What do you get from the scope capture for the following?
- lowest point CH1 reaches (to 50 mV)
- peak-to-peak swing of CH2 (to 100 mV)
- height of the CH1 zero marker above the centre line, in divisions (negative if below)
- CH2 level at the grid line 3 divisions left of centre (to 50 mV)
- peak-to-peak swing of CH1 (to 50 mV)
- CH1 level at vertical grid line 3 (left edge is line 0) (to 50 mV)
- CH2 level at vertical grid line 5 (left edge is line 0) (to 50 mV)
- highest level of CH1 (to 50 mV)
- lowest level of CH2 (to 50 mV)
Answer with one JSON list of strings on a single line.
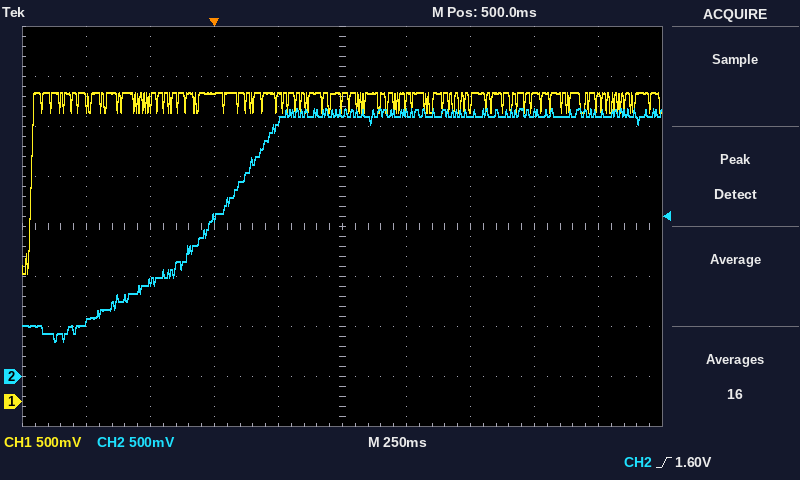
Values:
["1.30 V", "2.30 V", "-3.5 div", "950 mV", "1.80 V", "3.10 V", "2.65 V", "3.10 V", "350 mV"]
